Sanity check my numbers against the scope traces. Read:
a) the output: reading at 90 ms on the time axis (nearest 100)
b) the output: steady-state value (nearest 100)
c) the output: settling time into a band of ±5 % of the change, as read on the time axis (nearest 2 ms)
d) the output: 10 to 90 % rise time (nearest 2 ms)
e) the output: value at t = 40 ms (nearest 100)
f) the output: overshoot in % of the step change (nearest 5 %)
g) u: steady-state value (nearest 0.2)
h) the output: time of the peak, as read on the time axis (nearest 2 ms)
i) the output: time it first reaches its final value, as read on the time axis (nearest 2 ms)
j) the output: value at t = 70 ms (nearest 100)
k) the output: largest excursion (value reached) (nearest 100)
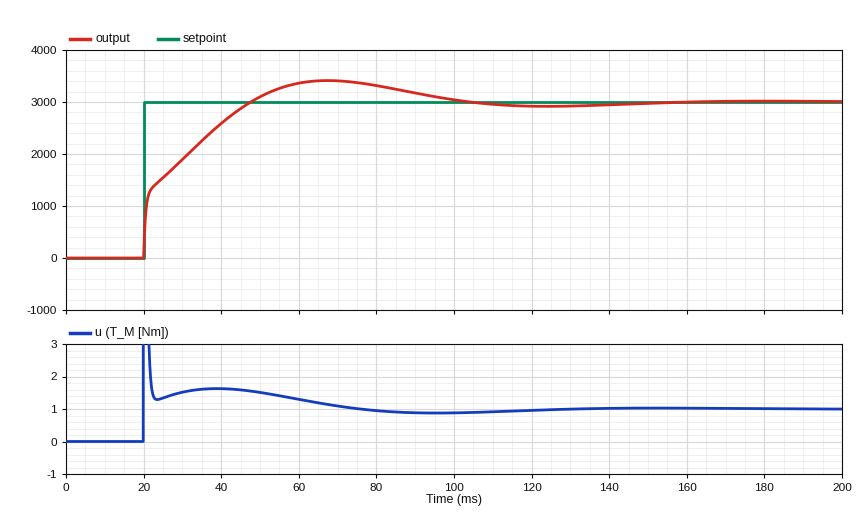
3200
3000
92 ms
22 ms
2600
15 %
1.0
68 ms
48 ms
3400
3400
